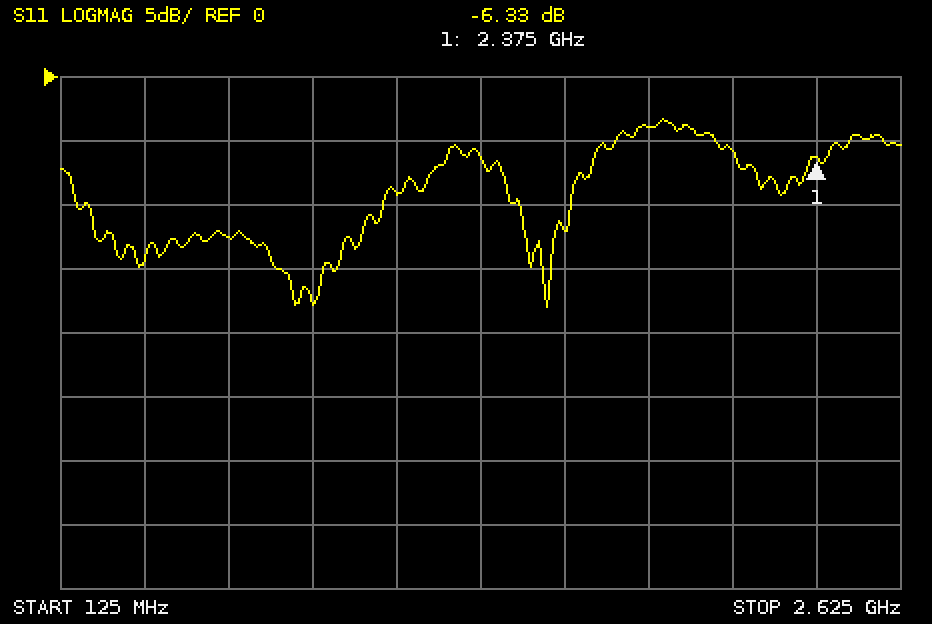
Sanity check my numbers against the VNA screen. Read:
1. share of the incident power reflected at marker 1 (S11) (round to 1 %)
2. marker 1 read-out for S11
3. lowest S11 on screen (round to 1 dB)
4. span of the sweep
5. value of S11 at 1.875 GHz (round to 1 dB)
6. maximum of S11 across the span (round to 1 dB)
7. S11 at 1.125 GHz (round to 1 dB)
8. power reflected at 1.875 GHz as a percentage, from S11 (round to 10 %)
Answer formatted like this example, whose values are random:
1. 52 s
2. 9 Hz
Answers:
1. 23 %
2. -6.33 dB
3. -18 dB
4. 2.5 GHz
5. -4 dB
6. -3 dB
7. -9 dB
8. 40 %
